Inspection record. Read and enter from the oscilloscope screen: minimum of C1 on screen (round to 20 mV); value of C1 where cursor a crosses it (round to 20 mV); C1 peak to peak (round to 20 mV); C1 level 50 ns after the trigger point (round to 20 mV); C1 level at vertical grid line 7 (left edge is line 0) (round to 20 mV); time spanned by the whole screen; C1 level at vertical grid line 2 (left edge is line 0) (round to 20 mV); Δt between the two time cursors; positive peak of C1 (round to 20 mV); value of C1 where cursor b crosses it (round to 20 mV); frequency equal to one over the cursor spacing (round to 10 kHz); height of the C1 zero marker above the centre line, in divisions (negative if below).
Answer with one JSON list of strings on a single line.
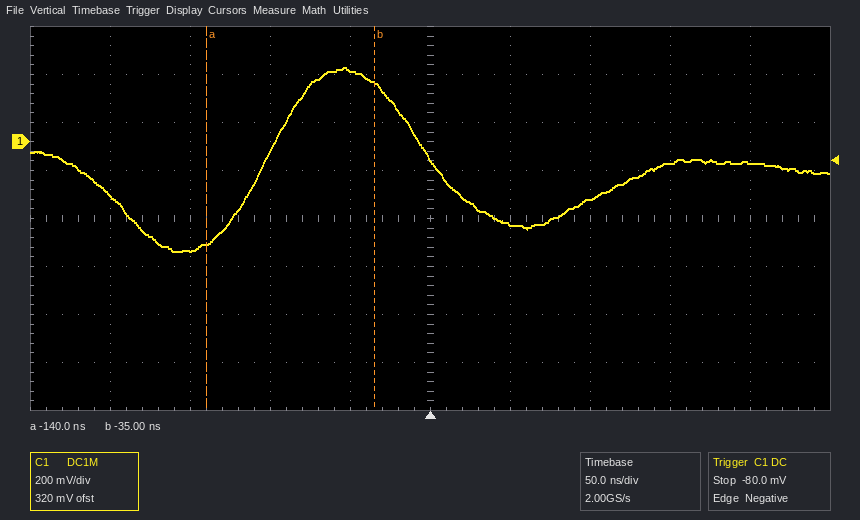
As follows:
["-460 mV", "-420 mV", "760 mV", "-340 mV", "-240 mV", "500 ns", "-460 mV", "105 ns", "300 mV", "240 mV", "9.52 MHz", "+1.6 div"]
